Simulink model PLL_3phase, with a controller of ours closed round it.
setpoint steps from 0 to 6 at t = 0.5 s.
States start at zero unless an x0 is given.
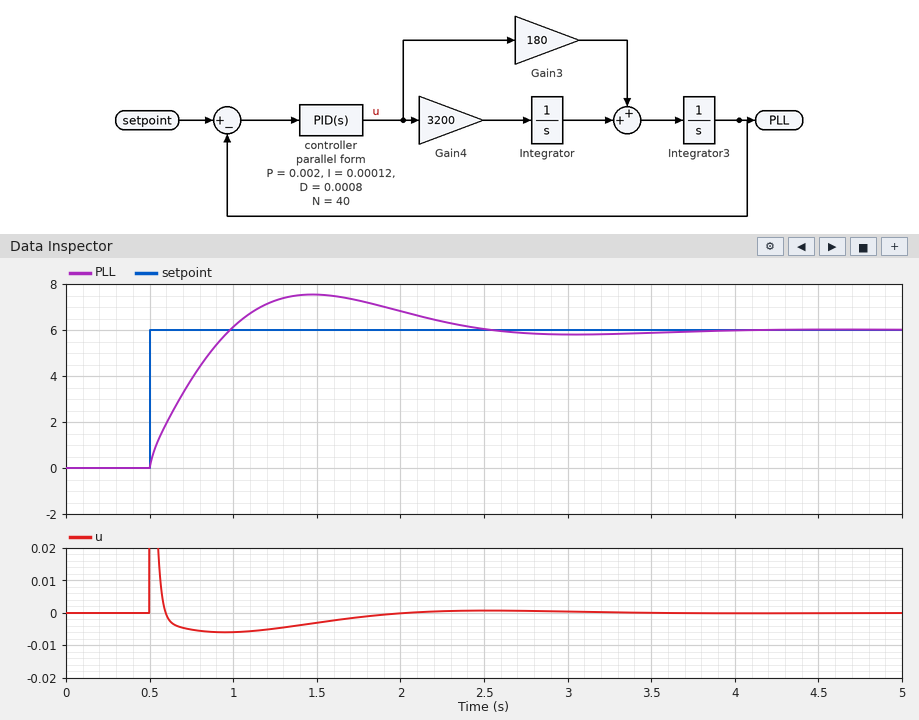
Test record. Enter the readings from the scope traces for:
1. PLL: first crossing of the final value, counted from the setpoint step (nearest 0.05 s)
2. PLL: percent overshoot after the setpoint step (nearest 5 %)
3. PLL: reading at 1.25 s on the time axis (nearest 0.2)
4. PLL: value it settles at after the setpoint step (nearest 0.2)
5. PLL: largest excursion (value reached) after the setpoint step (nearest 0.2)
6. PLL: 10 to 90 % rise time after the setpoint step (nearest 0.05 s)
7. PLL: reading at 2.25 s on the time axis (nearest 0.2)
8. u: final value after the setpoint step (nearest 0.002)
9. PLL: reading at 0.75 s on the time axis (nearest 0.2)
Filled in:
0.50 s
25 %
7.2
6.0
7.6
0.40 s
6.4
0.000
3.8
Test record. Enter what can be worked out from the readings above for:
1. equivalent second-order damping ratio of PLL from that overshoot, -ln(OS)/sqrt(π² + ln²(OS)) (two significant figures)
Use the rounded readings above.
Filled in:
0.40
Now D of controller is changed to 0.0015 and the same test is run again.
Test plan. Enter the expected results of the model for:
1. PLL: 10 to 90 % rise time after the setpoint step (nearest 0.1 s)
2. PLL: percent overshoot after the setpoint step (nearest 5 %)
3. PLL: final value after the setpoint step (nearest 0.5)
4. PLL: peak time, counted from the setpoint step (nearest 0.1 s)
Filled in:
0.3 s
15 %
6.0
0.9 s
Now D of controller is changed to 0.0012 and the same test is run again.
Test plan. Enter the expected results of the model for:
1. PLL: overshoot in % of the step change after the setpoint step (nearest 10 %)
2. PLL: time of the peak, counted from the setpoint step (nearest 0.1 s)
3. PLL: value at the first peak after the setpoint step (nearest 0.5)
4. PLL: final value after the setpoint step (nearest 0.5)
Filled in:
20 %
0.9 s
7.0
6.0
